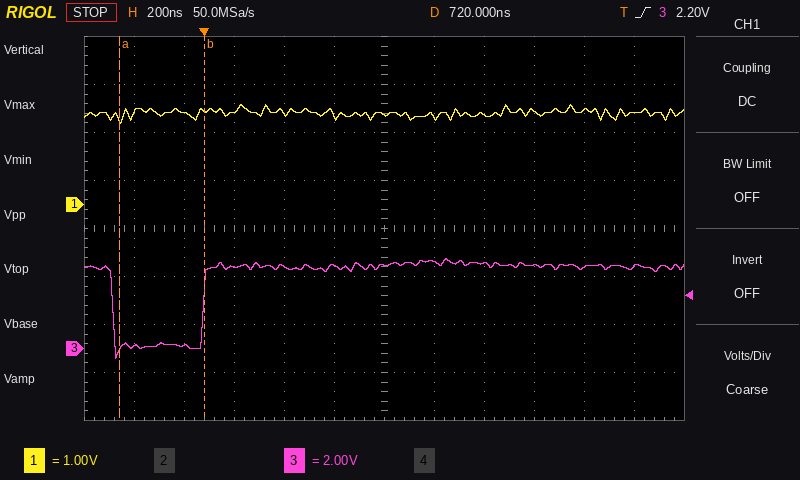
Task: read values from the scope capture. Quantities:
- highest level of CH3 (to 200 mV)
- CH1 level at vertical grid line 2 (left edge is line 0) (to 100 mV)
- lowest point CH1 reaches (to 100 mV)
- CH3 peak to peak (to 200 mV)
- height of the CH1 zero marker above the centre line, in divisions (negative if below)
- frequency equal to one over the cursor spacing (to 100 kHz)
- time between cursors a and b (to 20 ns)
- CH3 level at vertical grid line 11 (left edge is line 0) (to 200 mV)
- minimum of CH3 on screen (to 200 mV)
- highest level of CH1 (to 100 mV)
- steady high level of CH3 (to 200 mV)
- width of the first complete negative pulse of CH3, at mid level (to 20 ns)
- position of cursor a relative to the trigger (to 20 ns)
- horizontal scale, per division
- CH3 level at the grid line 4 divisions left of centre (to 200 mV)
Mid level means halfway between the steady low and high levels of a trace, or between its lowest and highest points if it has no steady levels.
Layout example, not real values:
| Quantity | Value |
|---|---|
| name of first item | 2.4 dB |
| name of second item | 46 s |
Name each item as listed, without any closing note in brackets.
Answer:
| Quantity | Value |
|---|---|
| highest level of CH3 | 3.8 V |
| CH1 level at vertical grid line 2 (left edge is line 0) | 1.9 V |
| lowest point CH1 reaches | 1.7 V |
| CH3 peak to peak | 4.2 V |
| height of the CH1 zero marker above the centre line, in divisions | +0.5 div |
| frequency equal to one over the cursor spacing | 2.9 MHz |
| time between cursors a and b | 340 ns |
| CH3 level at vertical grid line 11 (left edge is line 0) | 3.4 V |
| minimum of CH3 on screen | -400 mV |
| highest level of CH1 | 2.1 V |
| steady high level of CH3 | 3.4 V |
| width of the first complete negative pulse of CH3, at mid level | 360 ns |
| position of cursor a relative to the trigger | -340 ns |
| horizontal scale, per division | 200 ns |
| CH3 level at the grid line 4 divisions left of centre | 200 mV |
